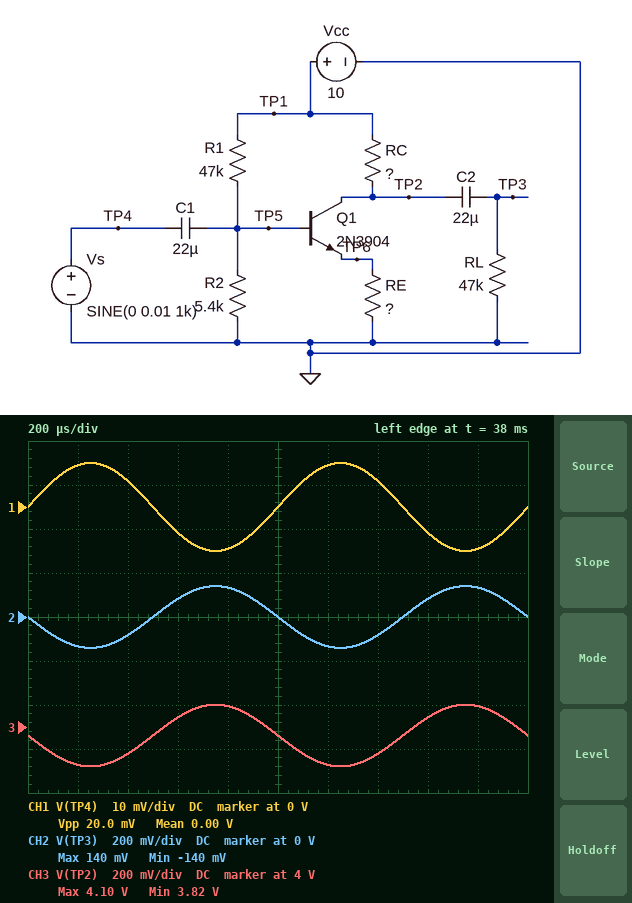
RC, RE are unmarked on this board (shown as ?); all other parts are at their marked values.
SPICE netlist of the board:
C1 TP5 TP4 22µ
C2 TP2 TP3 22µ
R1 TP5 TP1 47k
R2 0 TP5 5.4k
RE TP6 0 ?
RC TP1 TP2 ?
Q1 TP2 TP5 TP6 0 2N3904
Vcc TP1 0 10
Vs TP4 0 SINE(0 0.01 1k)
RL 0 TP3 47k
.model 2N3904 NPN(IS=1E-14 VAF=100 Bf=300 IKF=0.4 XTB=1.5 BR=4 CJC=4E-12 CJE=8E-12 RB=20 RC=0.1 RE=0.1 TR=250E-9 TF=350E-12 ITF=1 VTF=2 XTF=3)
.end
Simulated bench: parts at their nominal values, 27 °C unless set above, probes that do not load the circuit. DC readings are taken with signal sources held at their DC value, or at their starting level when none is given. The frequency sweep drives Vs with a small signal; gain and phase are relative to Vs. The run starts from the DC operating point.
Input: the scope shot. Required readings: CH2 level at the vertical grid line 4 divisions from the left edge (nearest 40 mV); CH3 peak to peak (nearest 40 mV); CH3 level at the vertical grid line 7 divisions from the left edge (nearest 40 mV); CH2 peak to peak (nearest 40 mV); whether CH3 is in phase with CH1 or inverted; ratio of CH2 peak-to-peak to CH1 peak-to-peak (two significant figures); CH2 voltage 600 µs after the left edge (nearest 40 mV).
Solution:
120 mV
280 mV
3.88 V
280 mV
inverted
14
80 mV
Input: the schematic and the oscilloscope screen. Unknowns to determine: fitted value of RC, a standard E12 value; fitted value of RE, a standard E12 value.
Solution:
5.6 kΩ
330 Ω
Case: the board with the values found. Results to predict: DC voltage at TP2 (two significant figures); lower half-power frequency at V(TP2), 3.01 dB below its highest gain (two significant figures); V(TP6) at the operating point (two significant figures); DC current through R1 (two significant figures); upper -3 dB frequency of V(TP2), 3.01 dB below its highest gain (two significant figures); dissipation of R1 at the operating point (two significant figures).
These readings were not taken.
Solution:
4.0 V
1.6 Hz
360 mV
190 µA
13 MHz
1.7 mW
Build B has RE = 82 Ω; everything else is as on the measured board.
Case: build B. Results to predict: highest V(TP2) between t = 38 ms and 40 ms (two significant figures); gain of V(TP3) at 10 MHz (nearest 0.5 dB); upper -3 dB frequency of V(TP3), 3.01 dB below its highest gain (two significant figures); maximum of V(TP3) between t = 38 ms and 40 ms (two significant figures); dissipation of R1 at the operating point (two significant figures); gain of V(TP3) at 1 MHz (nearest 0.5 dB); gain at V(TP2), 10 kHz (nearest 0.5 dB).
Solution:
450 mV
-1.5 dB
270 kHz
230 mV
1.8 mW
0.5 dB
9.5 dB
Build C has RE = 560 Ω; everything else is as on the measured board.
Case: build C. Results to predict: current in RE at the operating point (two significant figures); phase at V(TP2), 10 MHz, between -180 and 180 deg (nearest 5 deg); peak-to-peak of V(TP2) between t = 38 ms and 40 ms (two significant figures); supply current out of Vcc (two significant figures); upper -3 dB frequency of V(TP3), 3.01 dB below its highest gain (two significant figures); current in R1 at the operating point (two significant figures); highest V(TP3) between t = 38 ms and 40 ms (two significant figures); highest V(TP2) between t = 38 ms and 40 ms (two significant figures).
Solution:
670 µA
140 deg
170 mV
860 µA
16 MHz
190 µA
83 mV
6.3 V
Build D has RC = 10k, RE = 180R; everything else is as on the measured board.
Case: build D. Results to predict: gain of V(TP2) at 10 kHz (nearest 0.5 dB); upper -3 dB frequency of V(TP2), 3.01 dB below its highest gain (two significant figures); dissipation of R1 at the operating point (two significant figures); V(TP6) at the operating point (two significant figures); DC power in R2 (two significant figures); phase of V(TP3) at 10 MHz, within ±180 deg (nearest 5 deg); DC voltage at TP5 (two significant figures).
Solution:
2.5 dB
930 kHz
1.8 mW
180 mV
130 µW
5 deg
840 mV
